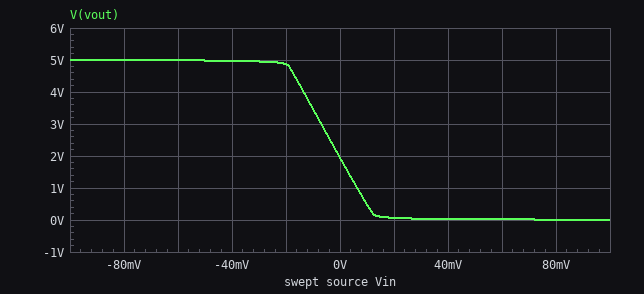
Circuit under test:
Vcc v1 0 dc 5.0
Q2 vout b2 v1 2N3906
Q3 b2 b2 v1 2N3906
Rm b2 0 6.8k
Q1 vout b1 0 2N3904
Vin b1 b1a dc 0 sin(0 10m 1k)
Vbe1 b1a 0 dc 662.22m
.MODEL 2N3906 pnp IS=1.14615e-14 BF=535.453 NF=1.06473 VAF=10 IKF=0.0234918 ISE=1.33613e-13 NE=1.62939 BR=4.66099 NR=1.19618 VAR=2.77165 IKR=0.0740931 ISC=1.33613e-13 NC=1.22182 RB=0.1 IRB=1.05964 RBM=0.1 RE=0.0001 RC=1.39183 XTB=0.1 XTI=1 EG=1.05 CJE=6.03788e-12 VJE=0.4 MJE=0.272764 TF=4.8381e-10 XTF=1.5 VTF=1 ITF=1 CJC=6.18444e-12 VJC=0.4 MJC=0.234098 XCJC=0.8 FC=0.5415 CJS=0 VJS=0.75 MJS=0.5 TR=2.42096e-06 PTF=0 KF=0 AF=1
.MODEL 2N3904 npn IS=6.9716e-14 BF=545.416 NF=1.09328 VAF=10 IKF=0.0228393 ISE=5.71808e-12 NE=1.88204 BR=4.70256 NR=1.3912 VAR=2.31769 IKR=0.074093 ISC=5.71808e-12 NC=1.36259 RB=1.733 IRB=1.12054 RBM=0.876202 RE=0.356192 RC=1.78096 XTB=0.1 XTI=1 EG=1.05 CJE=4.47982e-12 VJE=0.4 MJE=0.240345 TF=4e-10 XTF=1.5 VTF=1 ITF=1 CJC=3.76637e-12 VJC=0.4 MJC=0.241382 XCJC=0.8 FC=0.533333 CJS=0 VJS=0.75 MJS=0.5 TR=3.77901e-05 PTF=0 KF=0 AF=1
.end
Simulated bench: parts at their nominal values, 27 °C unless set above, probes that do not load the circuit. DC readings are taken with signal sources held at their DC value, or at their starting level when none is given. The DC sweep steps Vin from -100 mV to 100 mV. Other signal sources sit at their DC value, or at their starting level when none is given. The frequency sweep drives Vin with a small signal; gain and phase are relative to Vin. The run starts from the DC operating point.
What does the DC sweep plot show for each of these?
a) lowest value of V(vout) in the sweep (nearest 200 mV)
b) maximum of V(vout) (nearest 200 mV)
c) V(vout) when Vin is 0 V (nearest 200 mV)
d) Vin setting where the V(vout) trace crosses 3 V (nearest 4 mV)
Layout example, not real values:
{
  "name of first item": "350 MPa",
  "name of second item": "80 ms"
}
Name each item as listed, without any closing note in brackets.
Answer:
{
  "lowest value of V(vout) in the sweep": "0 V",
  "maximum of V(vout)": "5.0 V",
  "V(vout) when Vin is 0 V": "2.0 V",
  "Vin setting where the V(vout) trace crosses 3 V": "-8 mV"
}
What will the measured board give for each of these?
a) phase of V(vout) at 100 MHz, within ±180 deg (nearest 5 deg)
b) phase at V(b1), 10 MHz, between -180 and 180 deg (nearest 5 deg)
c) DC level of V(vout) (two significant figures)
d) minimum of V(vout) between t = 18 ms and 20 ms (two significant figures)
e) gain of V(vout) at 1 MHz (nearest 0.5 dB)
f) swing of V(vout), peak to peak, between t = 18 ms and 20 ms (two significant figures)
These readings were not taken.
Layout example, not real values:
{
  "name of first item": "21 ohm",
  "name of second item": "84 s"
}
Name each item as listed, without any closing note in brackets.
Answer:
{
  "phase of V(vout) at 100 MHz, within ±180 deg": "105 deg",
  "phase at V(b1), 10 MHz, between -180 and 180 deg": "0 deg",
  "DC level of V(vout)": "1.9 V",
  "minimum of V(vout) between t = 18 ms and 20 ms": "480 mV",
  "gain of V(vout) at 1 MHz": "43.0 dB",
  "swing of V(vout), peak to peak, between t = 18 ms and 20 ms": "3.0 V"
}
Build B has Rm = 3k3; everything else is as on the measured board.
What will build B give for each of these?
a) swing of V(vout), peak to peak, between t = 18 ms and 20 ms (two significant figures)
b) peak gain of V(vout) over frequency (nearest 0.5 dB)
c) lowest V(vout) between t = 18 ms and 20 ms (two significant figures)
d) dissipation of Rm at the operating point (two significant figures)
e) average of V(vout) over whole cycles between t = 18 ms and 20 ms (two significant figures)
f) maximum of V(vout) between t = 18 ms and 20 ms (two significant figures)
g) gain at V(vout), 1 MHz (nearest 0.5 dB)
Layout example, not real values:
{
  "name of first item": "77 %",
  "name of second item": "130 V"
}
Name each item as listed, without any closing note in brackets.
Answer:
{
  "swing of V(vout), peak to peak, between t = 18 ms and 20 ms": "1.2 V",
  "peak gain of V(vout) over frequency": "23.5 dB",
  "lowest V(vout) between t = 18 ms and 20 ms": "3.7 V",
  "dissipation of Rm at the operating point": "5.6 mW",
  "average of V(vout) over whole cycles between t = 18 ms and 20 ms": "4.6 V",
  "maximum of V(vout) between t = 18 ms and 20 ms": "5.0 V",
  "gain at V(vout), 1 MHz": "17.5 dB"
}
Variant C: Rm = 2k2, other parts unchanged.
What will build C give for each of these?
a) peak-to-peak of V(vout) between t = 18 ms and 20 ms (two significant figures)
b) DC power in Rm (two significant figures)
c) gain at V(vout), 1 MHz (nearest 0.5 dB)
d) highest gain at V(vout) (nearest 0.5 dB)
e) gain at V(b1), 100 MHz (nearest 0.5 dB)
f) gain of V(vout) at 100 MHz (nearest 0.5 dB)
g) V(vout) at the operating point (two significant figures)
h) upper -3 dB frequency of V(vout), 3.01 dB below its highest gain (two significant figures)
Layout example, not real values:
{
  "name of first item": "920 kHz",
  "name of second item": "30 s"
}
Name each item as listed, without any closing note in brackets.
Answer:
{
  "peak-to-peak of V(vout) between t = 18 ms and 20 ms": "55 mV",
  "DC power in Rm": "8.3 mW",
  "gain at V(vout), 1 MHz": "0.5 dB",
  "highest gain at V(vout)": "7.0 dB",
  "gain at V(b1), 100 MHz": "0 dB",
  "gain of V(vout) at 100 MHz": "-8.5 dB",
  "V(vout) at the operating point": "5.0 V",
  "upper -3 dB frequency of V(vout), 3.01 dB below its highest gain": "530 kHz"
}
